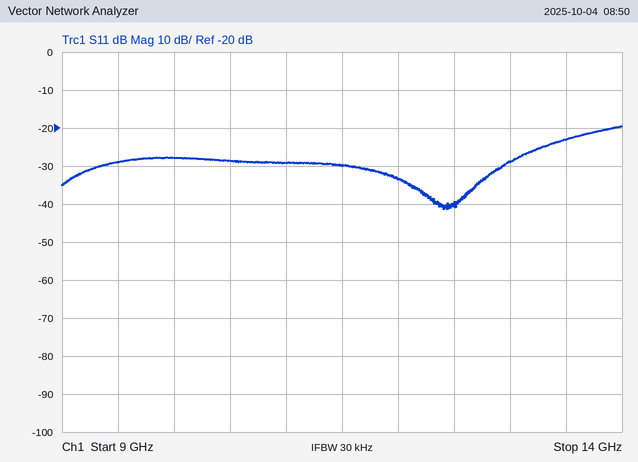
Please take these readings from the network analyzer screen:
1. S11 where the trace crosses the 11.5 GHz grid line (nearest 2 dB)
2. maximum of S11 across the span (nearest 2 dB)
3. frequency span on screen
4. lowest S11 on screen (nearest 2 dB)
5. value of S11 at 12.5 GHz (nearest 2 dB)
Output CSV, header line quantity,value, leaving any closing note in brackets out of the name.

quantity,value
S11 where the trace crosses the 11.5 GHz grid line,-30 dB
maximum of S11 across the span,-20 dB
frequency span on screen,5 GHz
lowest S11 on screen,-42 dB
value of S11 at 12.5 GHz,-40 dB
